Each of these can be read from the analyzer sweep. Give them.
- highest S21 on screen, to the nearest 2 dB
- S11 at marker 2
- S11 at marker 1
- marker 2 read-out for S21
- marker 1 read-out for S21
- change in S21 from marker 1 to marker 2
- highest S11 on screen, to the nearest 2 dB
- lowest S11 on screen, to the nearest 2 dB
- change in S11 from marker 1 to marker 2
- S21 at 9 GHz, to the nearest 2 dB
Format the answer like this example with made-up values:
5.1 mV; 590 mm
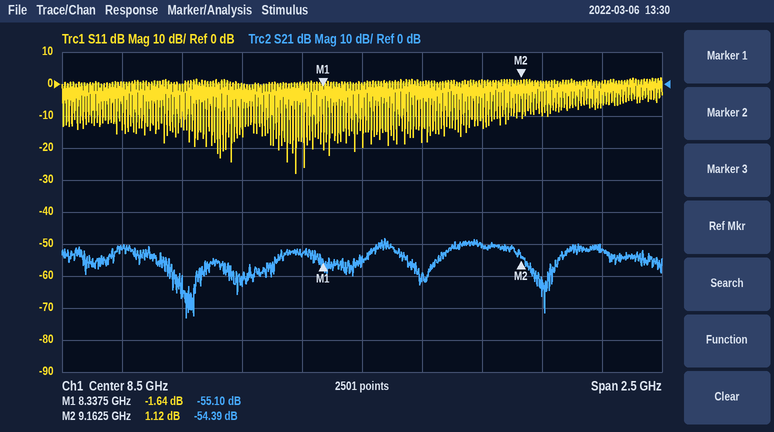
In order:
-48 dB; 1.12 dB; -1.64 dB; -54.39 dB; -55.10 dB; 0.71 dB; 2 dB; -28 dB; 2.76 dB; -50 dB
